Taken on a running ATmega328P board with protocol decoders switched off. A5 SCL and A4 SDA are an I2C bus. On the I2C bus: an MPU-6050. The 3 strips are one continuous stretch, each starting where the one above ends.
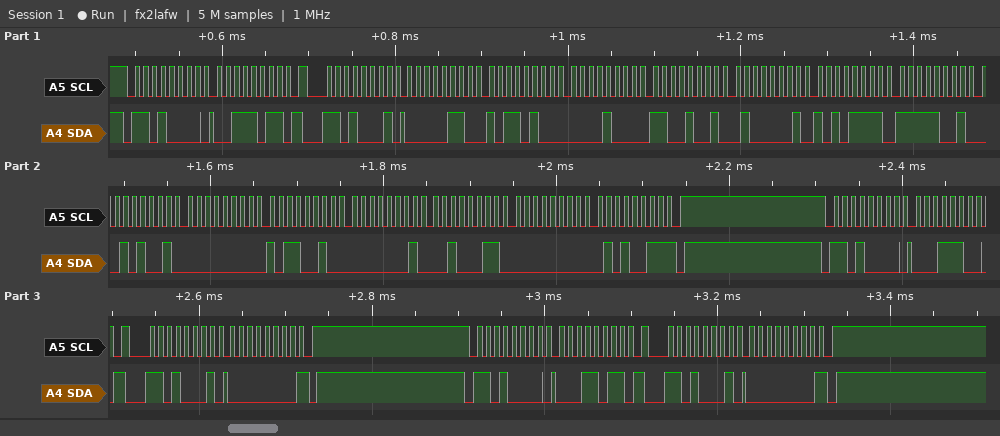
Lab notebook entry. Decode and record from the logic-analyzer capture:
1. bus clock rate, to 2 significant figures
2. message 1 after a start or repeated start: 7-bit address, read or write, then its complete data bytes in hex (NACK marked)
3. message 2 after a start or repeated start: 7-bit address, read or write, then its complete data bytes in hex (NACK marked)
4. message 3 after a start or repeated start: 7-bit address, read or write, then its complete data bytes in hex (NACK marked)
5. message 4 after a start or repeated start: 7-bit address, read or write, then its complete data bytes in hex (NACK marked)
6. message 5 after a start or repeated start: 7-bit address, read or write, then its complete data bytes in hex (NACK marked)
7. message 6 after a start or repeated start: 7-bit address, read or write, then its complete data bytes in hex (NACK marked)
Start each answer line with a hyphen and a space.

- 100 kHz
- 0x68 write: 3B
- 0x68 read: 06 B4 08 C9 41 AF F9 29 00 B2 01 23 00 53 NACK
- 0x68 write: 1C
- 0x68 read: 00 NACK
- 0x68 write: 1B
- 0x68 read: 00 NACK
